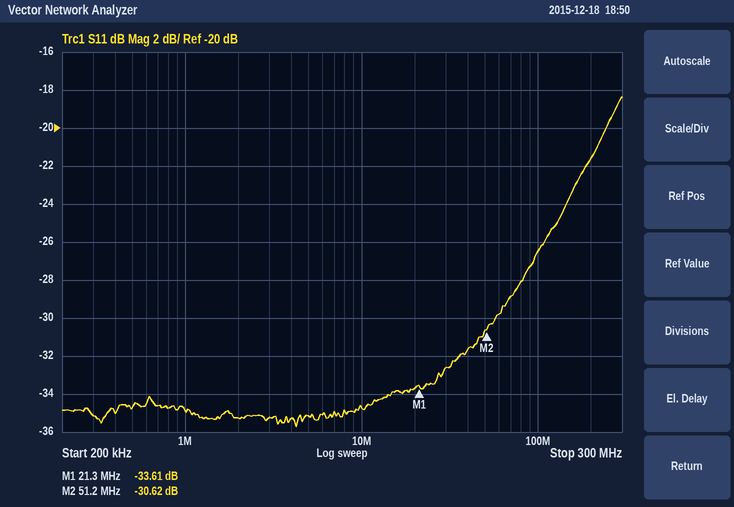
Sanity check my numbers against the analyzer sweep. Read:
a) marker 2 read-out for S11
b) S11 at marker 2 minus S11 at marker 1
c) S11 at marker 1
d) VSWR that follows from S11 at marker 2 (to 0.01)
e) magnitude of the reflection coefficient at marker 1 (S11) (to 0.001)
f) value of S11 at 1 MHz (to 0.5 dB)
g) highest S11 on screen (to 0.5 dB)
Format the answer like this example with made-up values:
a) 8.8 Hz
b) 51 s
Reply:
a) -30.62 dB
b) 2.99 dB
c) -33.61 dB
d) 1.06
e) 0.021
f) -35.0 dB
g) -18.5 dB
